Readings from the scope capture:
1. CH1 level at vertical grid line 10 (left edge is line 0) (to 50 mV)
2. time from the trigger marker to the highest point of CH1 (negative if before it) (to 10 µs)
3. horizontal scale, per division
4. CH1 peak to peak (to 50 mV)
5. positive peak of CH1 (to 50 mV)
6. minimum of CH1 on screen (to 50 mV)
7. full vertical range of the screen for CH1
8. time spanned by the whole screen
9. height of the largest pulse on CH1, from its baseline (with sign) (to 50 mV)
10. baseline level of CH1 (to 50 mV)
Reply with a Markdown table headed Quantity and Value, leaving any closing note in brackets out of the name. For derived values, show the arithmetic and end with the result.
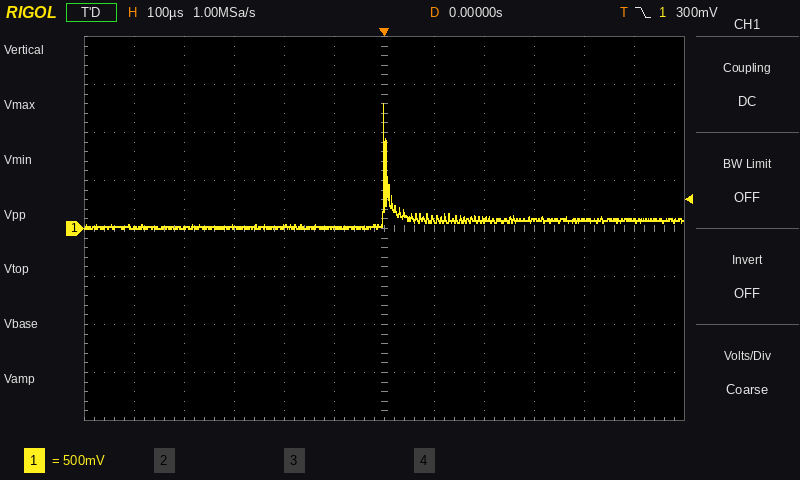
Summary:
| Quantity | Value |
|---|---|
| CH1 level at vertical grid line 10 (left edge is line 0) | 100 mV |
| time from the trigger marker to the highest point of CH1 (negative if before it) | 0 µs |
| horizontal scale, per division | 100 µs |
| CH1 peak to peak | 1.30 V − (0 mV) = 1.30 V |
| positive peak of CH1 | 1.30 V |
| minimum of CH1 on screen | 0 mV |
| full vertical range of the screen for CH1 | 4 V |
| time spanned by the whole screen | 1.2 ms |
| height of the largest pulse on CH1, from its baseline (with sign) | 1.30 V − (50 mV) = +1.25 V |
| baseline level of CH1 | 50 mV |
